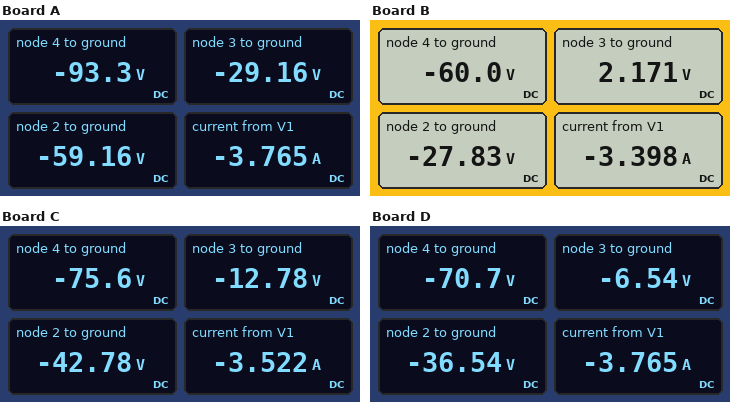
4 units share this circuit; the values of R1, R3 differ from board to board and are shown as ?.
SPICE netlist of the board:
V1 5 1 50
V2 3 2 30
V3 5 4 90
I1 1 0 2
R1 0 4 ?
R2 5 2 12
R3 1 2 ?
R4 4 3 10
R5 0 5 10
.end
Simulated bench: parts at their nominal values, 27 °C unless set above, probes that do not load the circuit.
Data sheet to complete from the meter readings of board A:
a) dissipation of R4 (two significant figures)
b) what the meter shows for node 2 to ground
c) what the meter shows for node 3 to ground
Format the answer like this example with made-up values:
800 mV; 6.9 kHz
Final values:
410 W; -59.16 V; -29.16 V
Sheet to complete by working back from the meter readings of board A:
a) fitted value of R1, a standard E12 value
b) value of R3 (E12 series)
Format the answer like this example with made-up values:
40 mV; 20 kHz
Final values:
56 Ω; 3.3 Ω
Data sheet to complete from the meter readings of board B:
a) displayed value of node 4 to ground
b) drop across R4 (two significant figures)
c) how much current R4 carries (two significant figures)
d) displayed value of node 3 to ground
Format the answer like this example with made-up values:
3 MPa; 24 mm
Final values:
-60.0 V; 62 V; 6.2 A; 2.171 V
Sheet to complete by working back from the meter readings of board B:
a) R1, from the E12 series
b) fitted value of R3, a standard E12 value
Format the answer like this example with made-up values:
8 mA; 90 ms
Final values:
12 Ω; 5.6 Ω
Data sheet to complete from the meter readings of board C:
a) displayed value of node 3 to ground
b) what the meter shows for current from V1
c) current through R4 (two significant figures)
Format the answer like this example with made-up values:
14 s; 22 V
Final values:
-12.78 V; -3.522 A; 6.3 A
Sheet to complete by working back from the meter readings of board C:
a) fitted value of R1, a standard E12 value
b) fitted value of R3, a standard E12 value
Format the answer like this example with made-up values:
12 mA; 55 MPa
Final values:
22 Ω; 4.7 Ω
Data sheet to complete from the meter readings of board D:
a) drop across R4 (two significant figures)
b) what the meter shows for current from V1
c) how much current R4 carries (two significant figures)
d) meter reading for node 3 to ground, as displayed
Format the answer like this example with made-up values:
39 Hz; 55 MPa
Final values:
64 V; -3.765 A; 6.4 A; -6.54 V
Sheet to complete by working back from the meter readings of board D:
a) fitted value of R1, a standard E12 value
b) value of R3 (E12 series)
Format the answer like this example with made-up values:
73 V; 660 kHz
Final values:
18 Ω; 3.3 Ω
